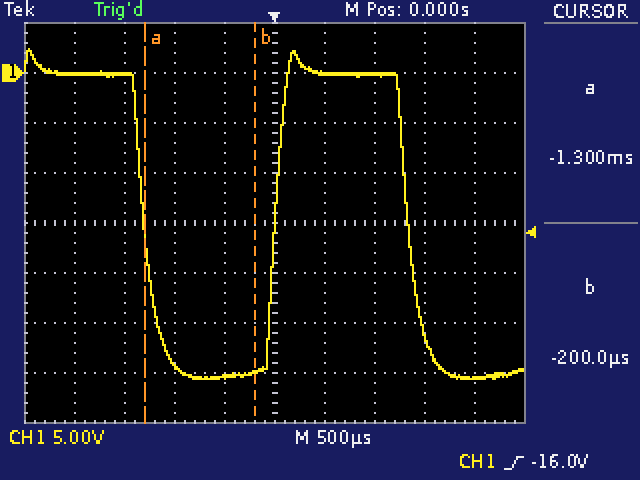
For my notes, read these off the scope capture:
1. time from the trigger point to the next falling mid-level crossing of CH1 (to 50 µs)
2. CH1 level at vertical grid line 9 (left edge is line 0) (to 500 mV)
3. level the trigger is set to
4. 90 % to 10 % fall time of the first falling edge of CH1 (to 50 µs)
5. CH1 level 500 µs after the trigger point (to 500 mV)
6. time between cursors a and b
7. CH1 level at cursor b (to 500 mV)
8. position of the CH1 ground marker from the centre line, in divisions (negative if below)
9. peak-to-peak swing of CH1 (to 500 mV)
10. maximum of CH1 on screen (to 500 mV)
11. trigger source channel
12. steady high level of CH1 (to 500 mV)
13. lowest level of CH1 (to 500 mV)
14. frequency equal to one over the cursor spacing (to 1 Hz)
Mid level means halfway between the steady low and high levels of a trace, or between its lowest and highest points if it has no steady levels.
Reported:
1.35 ms
-30.5 V
-16.0 V
300 µs
0.0 V
1.10 ms
-30.0 V
+3.0 div
33.0 V
2.5 V
CH1
0.0 V
-30.5 V
909 Hz
